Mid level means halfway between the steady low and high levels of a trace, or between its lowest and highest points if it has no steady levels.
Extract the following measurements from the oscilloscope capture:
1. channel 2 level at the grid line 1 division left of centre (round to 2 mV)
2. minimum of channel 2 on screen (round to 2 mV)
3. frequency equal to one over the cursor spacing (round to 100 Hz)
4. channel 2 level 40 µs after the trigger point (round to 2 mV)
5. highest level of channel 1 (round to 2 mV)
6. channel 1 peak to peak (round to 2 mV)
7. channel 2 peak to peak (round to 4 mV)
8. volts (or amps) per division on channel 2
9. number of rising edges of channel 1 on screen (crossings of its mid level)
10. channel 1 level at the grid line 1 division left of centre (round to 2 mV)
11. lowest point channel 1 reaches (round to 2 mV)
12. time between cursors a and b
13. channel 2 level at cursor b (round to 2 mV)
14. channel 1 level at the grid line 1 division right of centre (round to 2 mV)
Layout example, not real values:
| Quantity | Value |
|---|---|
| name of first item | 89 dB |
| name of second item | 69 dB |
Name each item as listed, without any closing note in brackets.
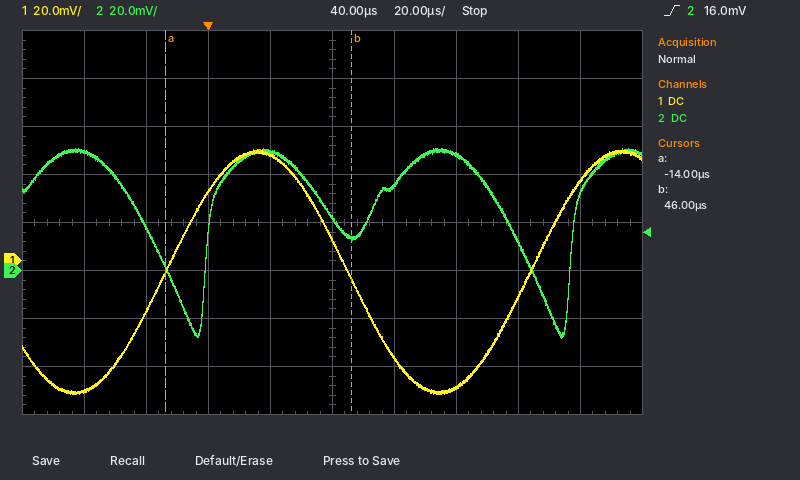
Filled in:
| Quantity | Value |
|---|---|
| channel 2 level at the grid line 1 division left of centre | 50 mV |
| minimum of channel 2 on screen | -28 mV |
| frequency equal to one over the cursor spacing | 16.7 kHz |
| channel 2 level 40 µs after the trigger point | 22 mV |
| highest level of channel 1 | 46 mV |
| channel 1 peak to peak | 102 mV |
| channel 2 peak to peak | 80 mV |
| volts (or amps) per division on channel 2 | 20 mV |
| number of rising edges of channel 1 on screen | 2 |
| channel 1 level at the grid line 1 division left of centre | 44 mV |
| lowest point channel 1 reaches | -56 mV |
| time between cursors a and b | 60 µs |
| channel 2 level at cursor b | 14 mV |
| channel 1 level at the grid line 1 division right of centre | -40 mV |
